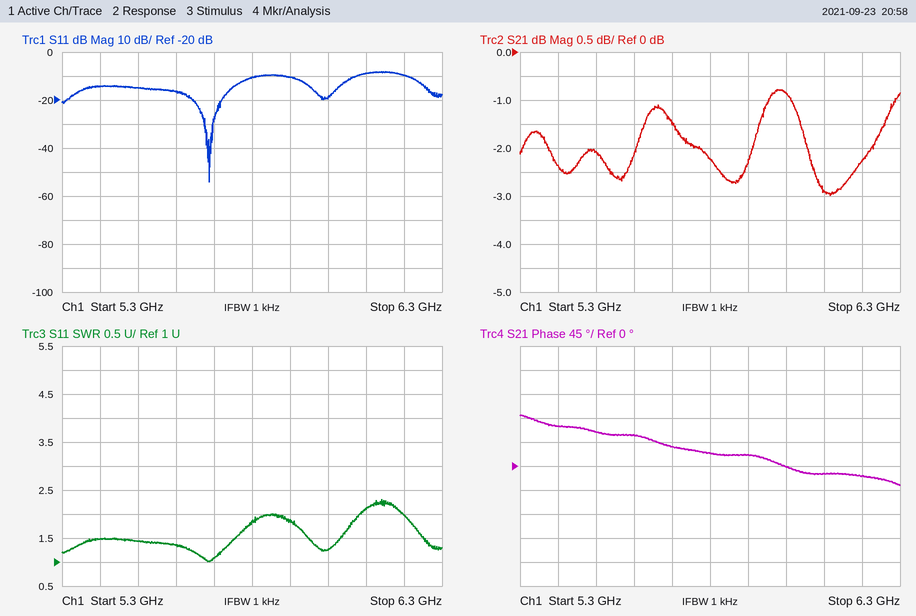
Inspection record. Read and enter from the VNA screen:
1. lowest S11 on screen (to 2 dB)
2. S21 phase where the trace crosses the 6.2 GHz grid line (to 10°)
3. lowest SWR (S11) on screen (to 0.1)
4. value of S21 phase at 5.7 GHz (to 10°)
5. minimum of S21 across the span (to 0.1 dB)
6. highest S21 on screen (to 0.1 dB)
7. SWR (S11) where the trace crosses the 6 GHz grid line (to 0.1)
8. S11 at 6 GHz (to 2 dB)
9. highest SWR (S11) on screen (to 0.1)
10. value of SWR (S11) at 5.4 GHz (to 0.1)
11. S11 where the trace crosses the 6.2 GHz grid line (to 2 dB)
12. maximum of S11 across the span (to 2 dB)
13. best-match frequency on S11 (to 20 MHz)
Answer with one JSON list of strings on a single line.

["-54 dB", "-20°", "1.0", "40°", "-3.0 dB", "-0.8 dB", "1.3", "-18 dB", "2.3", "1.5", "-10 dB", "-8 dB", "5.68 GHz"]
